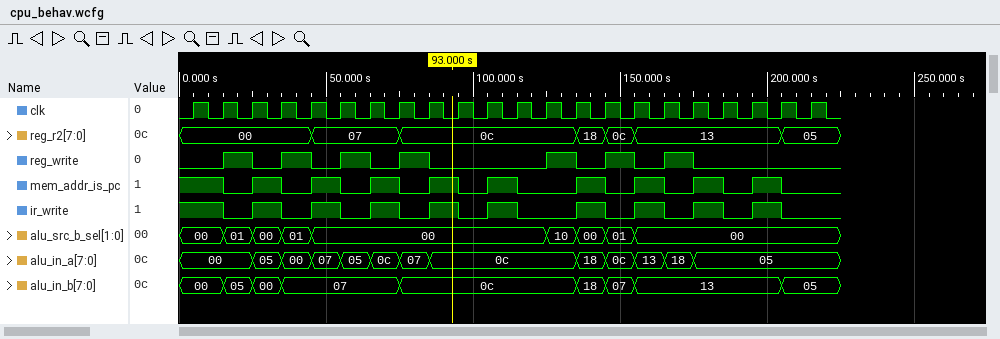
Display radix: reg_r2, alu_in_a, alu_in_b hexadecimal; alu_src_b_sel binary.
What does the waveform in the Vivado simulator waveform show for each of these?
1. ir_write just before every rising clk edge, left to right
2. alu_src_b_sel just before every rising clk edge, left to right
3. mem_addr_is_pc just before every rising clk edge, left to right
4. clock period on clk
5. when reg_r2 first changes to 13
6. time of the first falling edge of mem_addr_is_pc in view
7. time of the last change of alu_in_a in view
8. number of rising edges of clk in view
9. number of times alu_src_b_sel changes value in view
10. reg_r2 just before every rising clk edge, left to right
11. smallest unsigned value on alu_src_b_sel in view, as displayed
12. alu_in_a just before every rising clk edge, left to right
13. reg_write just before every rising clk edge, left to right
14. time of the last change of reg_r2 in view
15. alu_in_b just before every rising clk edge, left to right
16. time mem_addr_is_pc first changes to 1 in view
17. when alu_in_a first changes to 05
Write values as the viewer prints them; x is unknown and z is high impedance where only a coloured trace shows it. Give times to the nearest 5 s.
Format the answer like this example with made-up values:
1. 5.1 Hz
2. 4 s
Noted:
1. 1 1 0 1 0 1 0 1 0 1 0 1 0 0 1 0 1 0 1 0 1 0
2. 00, 00, 01, 00, 01, 00, 00, 00, 00, 00, 00, 00, 00, 10, 00, 01, 00, 00, 00, 00, 00, 00
3. 1 1 0 1 0 1 0 1 0 1 0 1 0 0 1 0 1 0 1 0 1 0
4. 10 s
5. 155 s
6. 15 s
7. 175 s
8. 22
9. 8
10. 00, 00, 00, 00, 00, 07, 07, 07, 0c, 0c, 0c, 0c, 0c, 0c, 18, 0c, 13, 13, 13, 13, 13, 05
11. 00
12. 00, 00, 00, 05, 00, 07, 05, 0c, 07, 0c, 0c, 0c, 0c, 0c, 18, 0c, 13, 18, 05, 05, 05, 05
13. 0 0 1 0 1 0 1 0 1 0 0 0 0 1 0 1 0 1 0 0 0 0
14. 205 s
15. 00, 00, 05, 00, 07, 07, 07, 07, 0c, 0c, 0c, 0c, 0c, 0c, 18, 07, 13, 13, 13, 13, 13, 05
16. 25 s
17. 25 s
